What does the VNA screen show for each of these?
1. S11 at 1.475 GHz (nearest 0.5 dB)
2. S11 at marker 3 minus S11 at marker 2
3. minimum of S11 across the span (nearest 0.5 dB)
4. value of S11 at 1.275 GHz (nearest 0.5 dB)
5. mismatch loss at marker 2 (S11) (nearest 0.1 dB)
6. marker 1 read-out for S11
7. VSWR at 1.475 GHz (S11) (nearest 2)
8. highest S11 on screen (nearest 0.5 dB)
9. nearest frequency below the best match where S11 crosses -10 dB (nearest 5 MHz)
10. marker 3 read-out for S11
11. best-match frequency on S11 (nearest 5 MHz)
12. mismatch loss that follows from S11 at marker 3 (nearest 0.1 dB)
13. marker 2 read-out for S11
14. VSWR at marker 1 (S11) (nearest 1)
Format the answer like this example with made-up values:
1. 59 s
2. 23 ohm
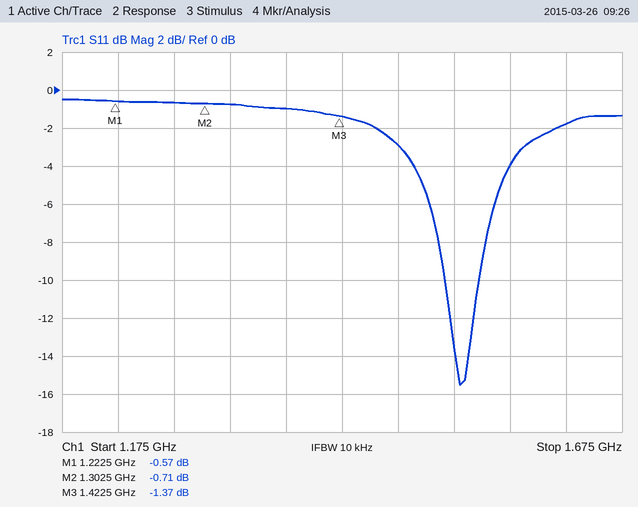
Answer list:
1. -3.0 dB
2. -0.66 dB
3. -15.5 dB
4. -0.5 dB
5. 8.2 dB
6. -0.57 dB
7. 6
8. -0.5 dB
9. 1.515 GHz
10. -1.37 dB
11. 1.530 GHz
12. 5.7 dB
13. -0.71 dB
14. 30
